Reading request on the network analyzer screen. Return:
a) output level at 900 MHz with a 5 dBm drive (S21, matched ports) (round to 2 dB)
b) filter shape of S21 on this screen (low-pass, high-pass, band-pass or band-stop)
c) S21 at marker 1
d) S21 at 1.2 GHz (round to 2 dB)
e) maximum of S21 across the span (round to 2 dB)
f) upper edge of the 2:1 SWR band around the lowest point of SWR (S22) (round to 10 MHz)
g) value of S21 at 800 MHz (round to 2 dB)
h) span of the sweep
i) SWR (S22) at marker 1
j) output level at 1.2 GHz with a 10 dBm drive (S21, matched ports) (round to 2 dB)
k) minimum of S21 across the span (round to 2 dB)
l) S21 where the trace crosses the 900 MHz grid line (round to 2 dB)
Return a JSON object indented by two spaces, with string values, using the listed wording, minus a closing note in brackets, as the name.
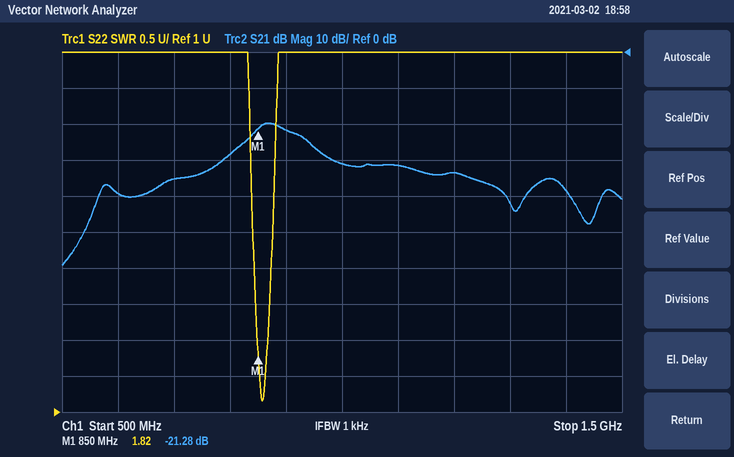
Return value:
{
  "output level at 900 MHz with a 5 dBm drive (S21, matched ports)": "-16 dBm",
  "filter shape of S21 on this screen": "band-pass",
  "S21 at marker 1": "-21.28 dB",
  "S21 at 1.2 GHz": "-34 dB",
  "maximum of S21 across the span": "-20 dB",
  "upper edge of the 2:1 SWR band around the lowest point of SWR (S22)": "870 MHz",
  "value of S21 at 800 MHz": "-28 dB",
  "span of the sweep": "1 GHz",
  "SWR (S22) at marker 1": "1.82",
  "output level at 1.2 GHz with a 10 dBm drive (S21, matched ports)": "-24 dBm",
  "minimum of S21 across the span": "-60 dB",
  "S21 where the trace crosses the 900 MHz grid line": "-22 dB"
}
